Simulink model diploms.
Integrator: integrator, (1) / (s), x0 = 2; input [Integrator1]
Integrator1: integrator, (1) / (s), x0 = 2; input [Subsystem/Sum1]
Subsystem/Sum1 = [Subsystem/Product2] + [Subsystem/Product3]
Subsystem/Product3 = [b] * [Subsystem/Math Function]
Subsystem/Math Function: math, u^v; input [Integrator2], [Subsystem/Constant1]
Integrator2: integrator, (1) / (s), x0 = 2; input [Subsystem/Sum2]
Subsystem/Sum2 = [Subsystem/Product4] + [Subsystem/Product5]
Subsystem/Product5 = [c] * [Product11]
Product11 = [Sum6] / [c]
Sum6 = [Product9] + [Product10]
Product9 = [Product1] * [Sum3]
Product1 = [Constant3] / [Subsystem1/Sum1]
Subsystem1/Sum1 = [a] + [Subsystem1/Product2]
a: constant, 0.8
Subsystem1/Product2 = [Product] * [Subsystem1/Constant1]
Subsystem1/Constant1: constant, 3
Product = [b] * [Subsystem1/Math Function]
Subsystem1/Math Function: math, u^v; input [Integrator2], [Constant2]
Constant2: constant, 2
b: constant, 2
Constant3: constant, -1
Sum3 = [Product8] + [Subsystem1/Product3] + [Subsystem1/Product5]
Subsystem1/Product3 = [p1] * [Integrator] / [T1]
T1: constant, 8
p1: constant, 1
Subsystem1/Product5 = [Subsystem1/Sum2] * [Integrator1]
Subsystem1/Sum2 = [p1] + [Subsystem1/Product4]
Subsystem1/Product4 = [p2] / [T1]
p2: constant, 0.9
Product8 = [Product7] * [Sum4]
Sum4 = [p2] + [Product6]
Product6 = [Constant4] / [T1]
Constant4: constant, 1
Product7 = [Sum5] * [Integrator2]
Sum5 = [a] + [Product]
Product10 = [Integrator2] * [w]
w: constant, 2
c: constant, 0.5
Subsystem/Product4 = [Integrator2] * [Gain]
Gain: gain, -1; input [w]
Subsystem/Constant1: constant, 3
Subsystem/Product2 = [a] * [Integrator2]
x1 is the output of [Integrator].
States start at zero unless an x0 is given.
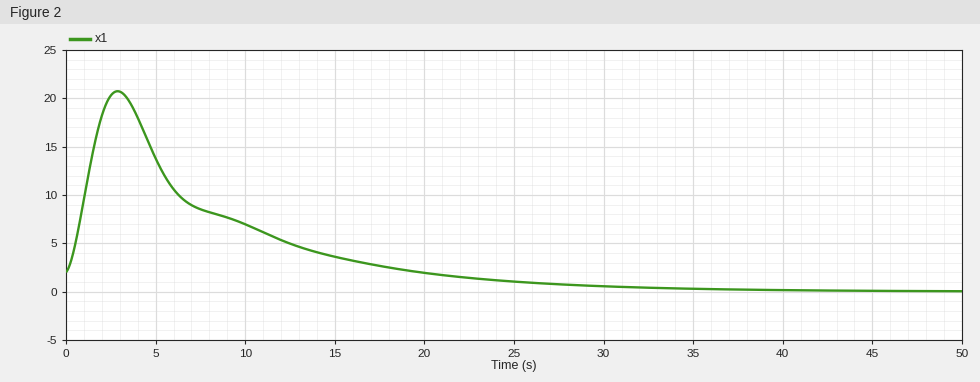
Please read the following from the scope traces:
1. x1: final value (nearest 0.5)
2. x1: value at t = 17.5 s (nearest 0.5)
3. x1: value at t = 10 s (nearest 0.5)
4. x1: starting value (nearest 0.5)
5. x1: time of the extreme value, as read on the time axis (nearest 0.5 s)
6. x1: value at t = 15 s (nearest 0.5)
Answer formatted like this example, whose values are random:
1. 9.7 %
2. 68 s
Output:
1. 0.0
2. 2.5
3. 7.0
4. 2.0
5. 3.0 s
6. 3.5
